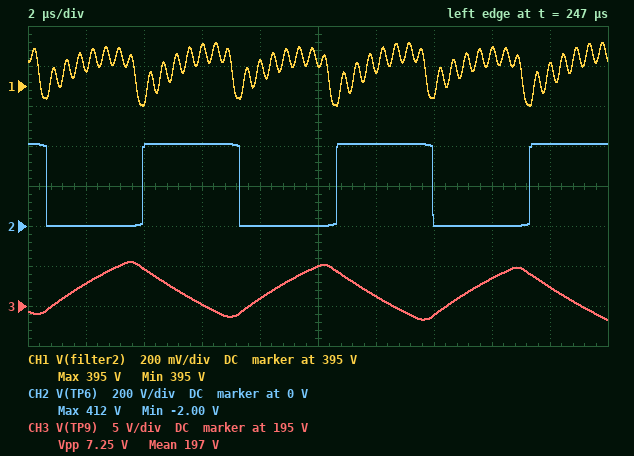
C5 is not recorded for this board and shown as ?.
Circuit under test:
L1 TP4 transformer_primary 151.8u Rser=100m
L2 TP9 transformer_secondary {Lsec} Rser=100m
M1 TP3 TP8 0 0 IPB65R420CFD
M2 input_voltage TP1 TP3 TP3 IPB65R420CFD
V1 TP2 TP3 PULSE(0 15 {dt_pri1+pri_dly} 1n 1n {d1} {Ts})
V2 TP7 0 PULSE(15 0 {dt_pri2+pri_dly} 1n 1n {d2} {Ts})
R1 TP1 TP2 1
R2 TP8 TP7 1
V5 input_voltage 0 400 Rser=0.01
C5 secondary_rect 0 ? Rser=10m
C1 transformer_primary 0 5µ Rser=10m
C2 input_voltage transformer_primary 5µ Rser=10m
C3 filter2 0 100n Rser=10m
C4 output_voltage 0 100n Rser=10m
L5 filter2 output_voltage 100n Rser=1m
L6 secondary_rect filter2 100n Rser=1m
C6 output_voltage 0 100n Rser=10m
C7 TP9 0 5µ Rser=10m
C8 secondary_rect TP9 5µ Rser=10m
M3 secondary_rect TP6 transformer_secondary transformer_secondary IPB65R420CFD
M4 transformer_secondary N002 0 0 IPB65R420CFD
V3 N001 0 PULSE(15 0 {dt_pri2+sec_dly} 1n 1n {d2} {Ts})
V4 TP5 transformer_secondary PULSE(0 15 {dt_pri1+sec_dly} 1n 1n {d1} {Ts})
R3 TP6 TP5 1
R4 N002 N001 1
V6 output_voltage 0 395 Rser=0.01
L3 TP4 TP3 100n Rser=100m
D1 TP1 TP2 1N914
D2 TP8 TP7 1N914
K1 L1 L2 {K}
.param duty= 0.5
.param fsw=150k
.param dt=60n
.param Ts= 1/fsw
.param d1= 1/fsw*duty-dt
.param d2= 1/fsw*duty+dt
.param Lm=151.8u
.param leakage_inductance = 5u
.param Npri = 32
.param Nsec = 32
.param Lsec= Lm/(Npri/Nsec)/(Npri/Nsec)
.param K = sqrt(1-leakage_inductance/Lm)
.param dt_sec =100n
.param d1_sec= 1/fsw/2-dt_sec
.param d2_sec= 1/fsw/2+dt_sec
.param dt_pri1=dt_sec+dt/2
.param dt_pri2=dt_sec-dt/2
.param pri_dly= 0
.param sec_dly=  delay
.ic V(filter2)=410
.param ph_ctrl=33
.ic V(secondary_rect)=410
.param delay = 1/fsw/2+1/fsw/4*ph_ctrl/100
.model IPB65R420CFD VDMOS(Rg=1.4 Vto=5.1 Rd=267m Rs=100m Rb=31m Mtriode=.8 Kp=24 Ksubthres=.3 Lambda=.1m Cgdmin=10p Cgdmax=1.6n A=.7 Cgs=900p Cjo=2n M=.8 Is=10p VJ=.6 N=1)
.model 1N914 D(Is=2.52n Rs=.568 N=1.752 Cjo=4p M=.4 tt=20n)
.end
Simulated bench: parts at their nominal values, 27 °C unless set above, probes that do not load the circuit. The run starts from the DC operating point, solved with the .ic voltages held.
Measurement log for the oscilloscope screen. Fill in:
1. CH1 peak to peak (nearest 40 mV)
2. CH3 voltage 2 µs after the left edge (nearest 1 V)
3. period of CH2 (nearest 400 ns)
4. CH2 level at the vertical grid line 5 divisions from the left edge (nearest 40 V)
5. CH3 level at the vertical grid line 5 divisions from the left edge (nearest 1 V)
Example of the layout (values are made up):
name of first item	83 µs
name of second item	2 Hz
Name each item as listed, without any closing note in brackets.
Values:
CH1 peak to peak	320 mV
CH3 voltage 2 µs after the left edge	198 V
period of CH2	6.8 µs
CH2 level at the vertical grid line 5 divisions from the left edge	0 V
CH3 level at the vertical grid line 5 divisions from the left edge	200 V
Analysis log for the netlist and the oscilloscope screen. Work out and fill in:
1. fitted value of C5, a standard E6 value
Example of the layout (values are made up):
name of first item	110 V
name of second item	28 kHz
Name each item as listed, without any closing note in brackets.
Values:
fitted value of C5, a standard E6 value	15 µF
